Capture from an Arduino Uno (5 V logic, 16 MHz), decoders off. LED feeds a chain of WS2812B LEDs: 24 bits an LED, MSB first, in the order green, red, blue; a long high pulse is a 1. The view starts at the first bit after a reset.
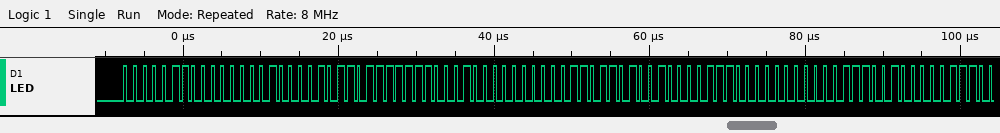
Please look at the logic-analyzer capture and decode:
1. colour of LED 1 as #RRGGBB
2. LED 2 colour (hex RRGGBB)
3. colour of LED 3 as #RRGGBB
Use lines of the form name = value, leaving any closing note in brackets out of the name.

colour of LED 1 as #RRGGBB = #01060B
LED 2 colour = #107F03
colour of LED 3 as #RRGGBB = #0E6900
